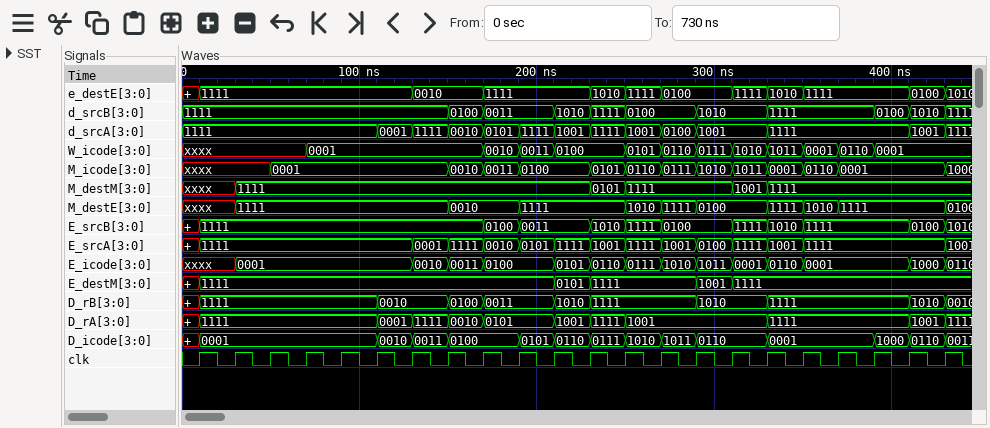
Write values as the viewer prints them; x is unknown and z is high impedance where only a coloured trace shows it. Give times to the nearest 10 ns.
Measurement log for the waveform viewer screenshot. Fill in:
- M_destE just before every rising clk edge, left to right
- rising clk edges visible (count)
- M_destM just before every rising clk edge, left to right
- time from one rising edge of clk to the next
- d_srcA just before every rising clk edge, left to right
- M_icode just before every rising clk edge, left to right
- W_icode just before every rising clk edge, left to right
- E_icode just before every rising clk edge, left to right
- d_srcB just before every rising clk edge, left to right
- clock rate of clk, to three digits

xxxx, xxxx, 1111, 1111, 1111, 1111, 1111, 1111, 0010, 0010, 1111, 1111, 1111, 1010, 1111, 0100, 0100, 1111, 1010, 1111, 1111, 1111
22
xxxx, xxxx, 1111, 1111, 1111, 1111, 1111, 1111, 1111, 1111, 1111, 1111, 0101, 1111, 1111, 1111, 1001, 1111, 1111, 1111, 1111, 1111
20 ns
1111, 1111, 1111, 1111, 1111, 1111, 0001, 1111, 0010, 0101, 1111, 1001, 1111, 1001, 0100, 1001, 1001, 1111, 1111, 1111, 1111, 1001
xxxx, xxxx, xxxx, 0001, 0001, 0001, 0001, 0001, 0010, 0011, 0100, 0100, 0101, 0110, 0111, 1010, 1011, 0001, 0110, 0001, 0001, 0001
xxxx, xxxx, xxxx, xxxx, 0001, 0001, 0001, 0001, 0001, 0010, 0011, 0100, 0100, 0101, 0110, 0111, 1010, 1011, 0001, 0110, 0001, 0001
xxxx, xxxx, 0001, 0001, 0001, 0001, 0001, 0010, 0011, 0100, 0100, 0101, 0110, 0111, 1010, 1011, 0001, 0110, 0001, 0001, 0001, 1000
1111, 1111, 1111, 1111, 1111, 1111, 1111, 1111, 0100, 0011, 0011, 1010, 1111, 0100, 0100, 1010, 1010, 1111, 1111, 1111, 0100, 1010
50.0 MHz
